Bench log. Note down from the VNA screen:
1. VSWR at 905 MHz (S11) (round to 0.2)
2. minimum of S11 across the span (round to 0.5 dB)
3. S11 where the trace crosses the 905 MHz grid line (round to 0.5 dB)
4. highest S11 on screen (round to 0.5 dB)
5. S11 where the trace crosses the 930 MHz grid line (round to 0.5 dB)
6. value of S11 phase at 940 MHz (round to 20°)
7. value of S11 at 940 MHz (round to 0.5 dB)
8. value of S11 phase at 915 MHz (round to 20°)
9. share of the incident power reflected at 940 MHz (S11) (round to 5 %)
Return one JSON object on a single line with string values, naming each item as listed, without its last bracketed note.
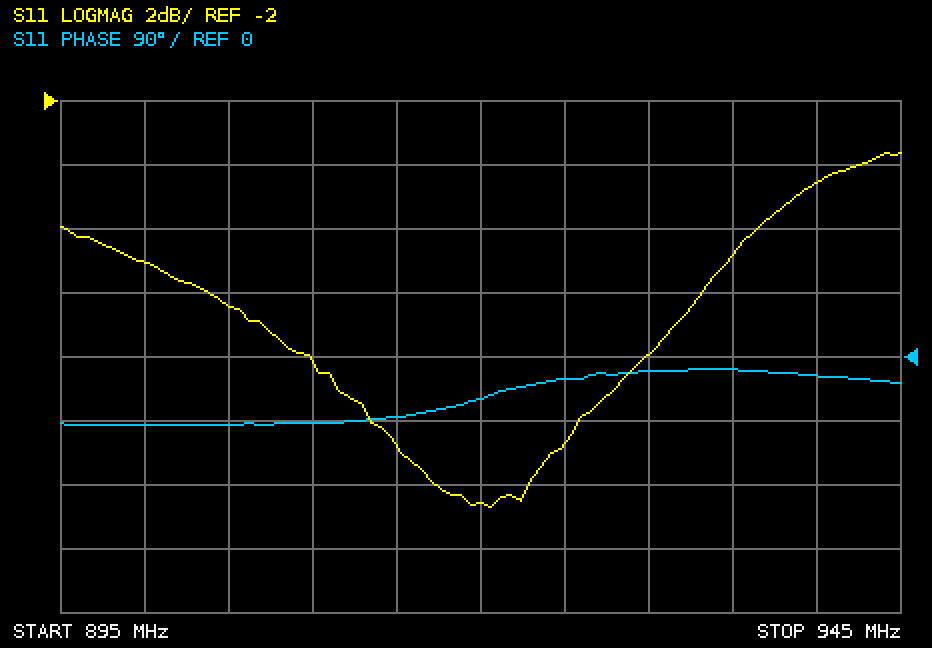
{"VSWR at 905 MHz (S11)": "2.2", "minimum of S11 across the span": "-14.5 dB", "S11 where the trace crosses the 905 MHz grid line": "-8.5 dB", "highest S11 on screen": "-3.5 dB", "S11 where the trace crosses the 930 MHz grid line": "-10.0 dB", "value of S11 phase at 940 MHz": "-20°", "value of S11 at 940 MHz": "-4.5 dB", "value of S11 phase at 915 MHz": "-80°", "share of the incident power reflected at 940 MHz (S11)": "35 %"}
